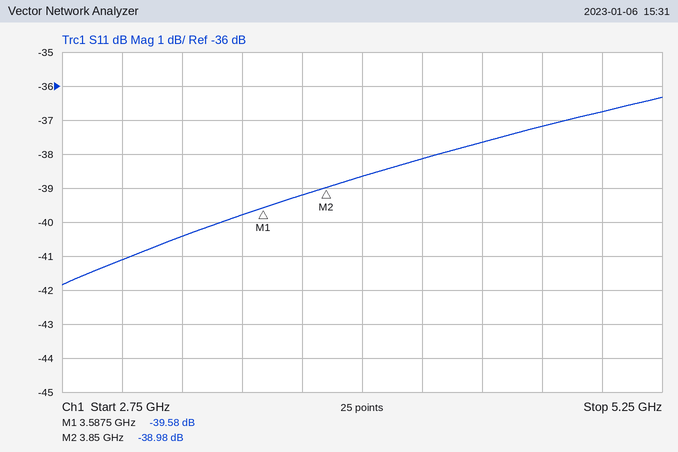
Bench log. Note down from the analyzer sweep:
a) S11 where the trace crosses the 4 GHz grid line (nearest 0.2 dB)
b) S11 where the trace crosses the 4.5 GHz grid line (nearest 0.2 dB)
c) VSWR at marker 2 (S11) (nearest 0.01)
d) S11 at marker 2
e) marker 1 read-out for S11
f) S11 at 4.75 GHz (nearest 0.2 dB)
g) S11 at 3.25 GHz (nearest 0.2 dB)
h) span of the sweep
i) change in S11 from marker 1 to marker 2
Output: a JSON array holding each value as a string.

["-38.6 dB", "-37.6 dB", "1.02", "-38.98 dB", "-39.58 dB", "-37.2 dB", "-40.4 dB", "2.5 GHz", "0.60 dB"]
